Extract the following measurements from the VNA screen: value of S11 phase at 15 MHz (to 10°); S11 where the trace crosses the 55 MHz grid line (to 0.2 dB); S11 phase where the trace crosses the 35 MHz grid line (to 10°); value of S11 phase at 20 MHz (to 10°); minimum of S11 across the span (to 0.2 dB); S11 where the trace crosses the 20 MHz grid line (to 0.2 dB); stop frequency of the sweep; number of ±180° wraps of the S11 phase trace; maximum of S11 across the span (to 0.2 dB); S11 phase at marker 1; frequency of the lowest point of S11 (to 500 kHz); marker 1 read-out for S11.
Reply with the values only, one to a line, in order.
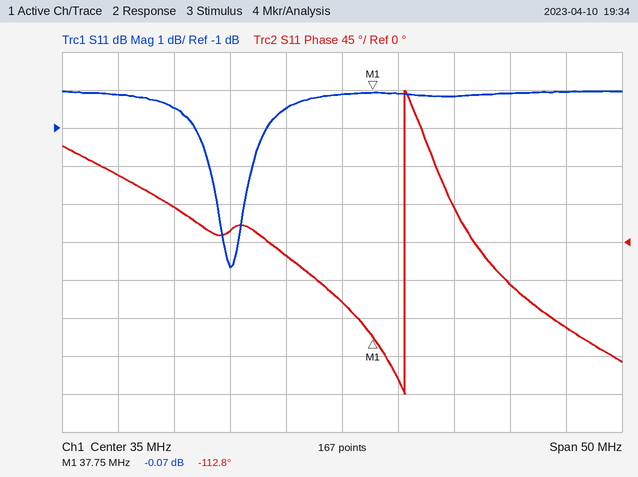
80°
0.0 dB
-70°
40°
-4.6 dB
-0.4 dB
60 MHz
1
0.0 dB
-112.8°
25.0 MHz
-0.07 dB
